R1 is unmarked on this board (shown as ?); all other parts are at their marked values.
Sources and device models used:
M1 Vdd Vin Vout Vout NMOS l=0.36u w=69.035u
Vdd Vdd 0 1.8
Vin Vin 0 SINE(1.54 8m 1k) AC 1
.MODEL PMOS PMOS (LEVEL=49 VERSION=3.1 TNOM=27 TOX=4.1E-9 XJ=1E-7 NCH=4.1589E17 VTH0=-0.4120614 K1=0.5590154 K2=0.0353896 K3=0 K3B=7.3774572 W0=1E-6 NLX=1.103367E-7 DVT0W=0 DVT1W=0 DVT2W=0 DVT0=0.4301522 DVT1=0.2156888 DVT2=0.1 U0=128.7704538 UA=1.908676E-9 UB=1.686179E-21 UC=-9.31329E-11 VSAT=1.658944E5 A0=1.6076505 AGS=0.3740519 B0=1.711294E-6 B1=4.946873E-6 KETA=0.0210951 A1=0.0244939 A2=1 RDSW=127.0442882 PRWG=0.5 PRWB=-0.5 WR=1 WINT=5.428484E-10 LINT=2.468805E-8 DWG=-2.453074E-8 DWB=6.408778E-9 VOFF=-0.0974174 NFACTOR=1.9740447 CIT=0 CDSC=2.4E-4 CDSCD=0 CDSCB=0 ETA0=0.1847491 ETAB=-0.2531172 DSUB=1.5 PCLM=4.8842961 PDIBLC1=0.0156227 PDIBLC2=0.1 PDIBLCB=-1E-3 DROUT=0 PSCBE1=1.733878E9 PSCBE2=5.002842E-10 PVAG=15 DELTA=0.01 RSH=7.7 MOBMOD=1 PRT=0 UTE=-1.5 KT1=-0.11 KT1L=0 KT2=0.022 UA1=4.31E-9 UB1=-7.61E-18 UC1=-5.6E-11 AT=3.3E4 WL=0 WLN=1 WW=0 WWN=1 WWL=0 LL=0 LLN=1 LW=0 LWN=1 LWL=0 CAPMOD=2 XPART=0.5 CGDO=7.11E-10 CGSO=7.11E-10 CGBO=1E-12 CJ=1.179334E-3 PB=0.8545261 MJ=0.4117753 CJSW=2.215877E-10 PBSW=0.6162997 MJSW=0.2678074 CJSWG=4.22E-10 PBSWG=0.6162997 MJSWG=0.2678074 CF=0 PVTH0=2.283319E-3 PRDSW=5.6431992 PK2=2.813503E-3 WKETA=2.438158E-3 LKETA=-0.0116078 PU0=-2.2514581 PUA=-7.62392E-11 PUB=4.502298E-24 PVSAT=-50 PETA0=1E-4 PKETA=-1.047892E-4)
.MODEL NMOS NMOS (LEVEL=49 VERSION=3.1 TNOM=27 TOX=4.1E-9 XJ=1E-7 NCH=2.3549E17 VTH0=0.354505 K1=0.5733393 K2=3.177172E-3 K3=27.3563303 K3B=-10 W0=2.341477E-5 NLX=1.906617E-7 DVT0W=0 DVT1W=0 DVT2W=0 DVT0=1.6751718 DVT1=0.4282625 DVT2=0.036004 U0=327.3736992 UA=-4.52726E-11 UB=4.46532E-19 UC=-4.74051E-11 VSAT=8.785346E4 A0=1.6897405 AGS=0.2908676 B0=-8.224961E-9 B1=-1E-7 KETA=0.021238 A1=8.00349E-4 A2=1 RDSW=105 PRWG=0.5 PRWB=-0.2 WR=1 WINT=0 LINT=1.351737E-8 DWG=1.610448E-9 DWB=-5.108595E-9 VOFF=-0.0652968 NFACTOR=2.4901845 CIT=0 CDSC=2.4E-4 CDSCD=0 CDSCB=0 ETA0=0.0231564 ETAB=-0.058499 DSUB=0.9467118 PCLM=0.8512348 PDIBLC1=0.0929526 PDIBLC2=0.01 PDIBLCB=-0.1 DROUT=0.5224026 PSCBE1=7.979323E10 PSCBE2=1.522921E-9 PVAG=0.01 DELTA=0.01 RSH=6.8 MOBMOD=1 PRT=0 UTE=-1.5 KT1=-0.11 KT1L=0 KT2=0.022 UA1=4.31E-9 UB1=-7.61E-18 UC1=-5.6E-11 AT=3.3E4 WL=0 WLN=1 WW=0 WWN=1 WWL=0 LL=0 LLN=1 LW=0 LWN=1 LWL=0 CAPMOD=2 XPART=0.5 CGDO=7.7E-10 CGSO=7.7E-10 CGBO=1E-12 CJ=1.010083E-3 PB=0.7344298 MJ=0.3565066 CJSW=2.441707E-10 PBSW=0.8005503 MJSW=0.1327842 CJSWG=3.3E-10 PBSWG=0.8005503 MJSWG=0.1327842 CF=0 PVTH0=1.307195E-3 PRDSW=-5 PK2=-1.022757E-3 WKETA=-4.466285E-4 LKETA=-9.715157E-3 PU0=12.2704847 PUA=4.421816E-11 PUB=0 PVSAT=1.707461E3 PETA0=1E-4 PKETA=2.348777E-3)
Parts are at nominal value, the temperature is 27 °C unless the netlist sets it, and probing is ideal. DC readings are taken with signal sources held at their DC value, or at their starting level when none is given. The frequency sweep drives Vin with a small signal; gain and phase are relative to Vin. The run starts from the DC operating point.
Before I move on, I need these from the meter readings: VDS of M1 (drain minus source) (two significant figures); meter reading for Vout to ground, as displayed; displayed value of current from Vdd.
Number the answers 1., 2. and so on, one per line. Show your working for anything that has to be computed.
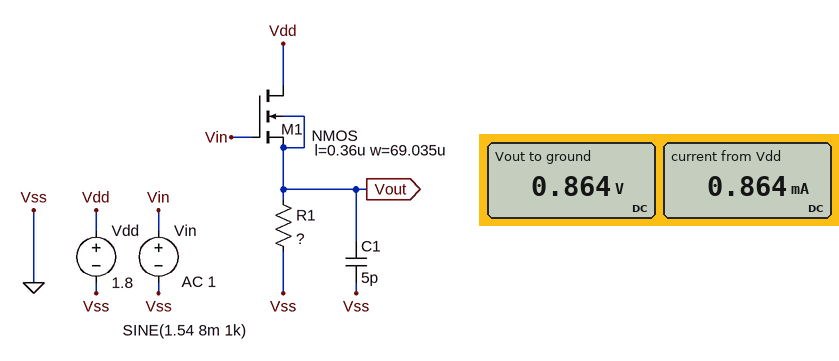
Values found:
1. 1.8 V - 864 mV = 940 mV
2. 0.864 V
3. 0.864 mA
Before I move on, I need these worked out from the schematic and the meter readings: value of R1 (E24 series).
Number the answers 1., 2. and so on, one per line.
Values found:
1. 1 kΩ
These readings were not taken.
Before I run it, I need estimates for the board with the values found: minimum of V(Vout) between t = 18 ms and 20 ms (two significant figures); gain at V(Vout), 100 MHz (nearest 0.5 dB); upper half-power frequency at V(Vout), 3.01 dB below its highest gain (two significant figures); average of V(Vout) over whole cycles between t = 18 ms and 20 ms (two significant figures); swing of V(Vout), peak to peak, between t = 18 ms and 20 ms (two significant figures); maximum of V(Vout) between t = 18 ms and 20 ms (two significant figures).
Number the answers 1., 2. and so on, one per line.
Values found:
1. 860 mV
2. -1.5 dB
3. 300 MHz
4. 860 mV
5. 14 mV
6. 870 mV
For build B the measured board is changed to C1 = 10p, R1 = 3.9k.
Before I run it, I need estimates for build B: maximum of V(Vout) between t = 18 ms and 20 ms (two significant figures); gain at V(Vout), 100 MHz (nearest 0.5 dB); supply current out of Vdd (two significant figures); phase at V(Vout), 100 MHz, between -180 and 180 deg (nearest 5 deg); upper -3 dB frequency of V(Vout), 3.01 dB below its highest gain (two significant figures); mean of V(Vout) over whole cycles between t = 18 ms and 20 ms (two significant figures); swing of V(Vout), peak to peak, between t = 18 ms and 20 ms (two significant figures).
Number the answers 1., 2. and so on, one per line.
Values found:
1. 970 mV
2. -5.5 dB
3. 250 µA
4. -55 deg
5. 69 MHz
6. 960 mV
7. 15 mV
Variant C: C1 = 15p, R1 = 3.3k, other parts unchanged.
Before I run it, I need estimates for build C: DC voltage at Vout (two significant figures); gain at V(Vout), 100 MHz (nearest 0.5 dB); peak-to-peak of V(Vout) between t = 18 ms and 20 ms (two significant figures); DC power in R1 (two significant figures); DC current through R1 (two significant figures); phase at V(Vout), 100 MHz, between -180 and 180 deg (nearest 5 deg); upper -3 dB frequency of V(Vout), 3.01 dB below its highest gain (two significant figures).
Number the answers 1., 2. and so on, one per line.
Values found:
1. 950 mV
2. -7.5 dB
3. 15 mV
4. 270 µW
5. 290 µA
6. -60 deg
7. 52 MHz
